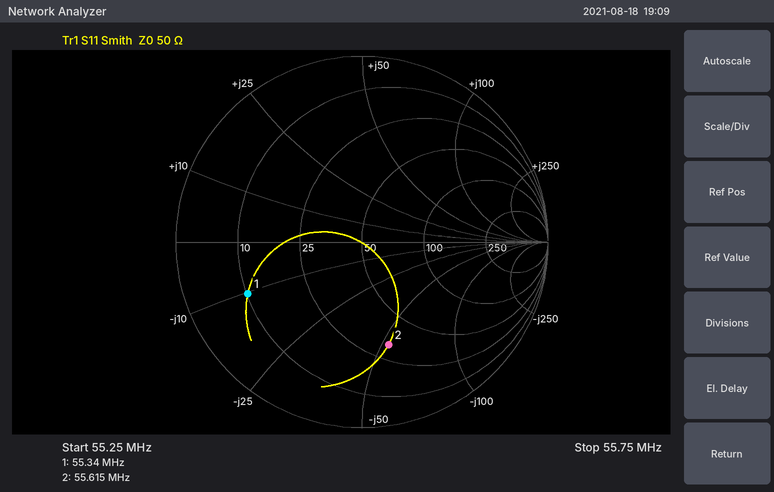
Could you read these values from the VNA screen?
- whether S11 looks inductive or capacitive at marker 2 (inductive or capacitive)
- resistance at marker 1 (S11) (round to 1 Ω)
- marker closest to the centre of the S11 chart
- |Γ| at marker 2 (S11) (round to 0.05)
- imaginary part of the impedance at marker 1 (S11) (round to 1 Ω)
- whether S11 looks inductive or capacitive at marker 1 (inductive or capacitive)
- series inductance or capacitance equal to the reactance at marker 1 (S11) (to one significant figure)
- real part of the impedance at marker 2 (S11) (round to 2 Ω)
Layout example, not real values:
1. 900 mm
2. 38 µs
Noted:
1. capacitive
2. 10 Ω
3. marker 2
4. 0.55
5. -10 Ω
6. capacitive
7. 300 pF
8. 32 Ω
